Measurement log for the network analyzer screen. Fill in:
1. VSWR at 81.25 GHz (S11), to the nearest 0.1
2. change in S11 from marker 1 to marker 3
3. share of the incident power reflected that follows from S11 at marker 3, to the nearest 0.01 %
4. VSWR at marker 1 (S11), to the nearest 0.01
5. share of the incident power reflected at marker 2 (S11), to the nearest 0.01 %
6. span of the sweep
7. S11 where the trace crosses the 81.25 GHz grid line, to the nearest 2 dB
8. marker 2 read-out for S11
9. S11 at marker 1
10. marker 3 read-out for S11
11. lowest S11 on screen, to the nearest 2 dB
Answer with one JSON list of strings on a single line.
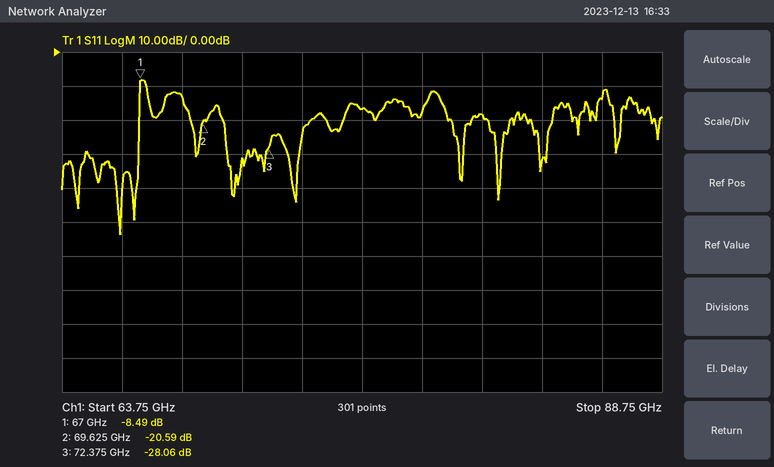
["1.3", "-19.57 dB", "0.16 %", "2.21", "0.87 %", "25 GHz", "-18 dB", "-20.59 dB", "-8.49 dB", "-28.06 dB", "-54 dB"]
